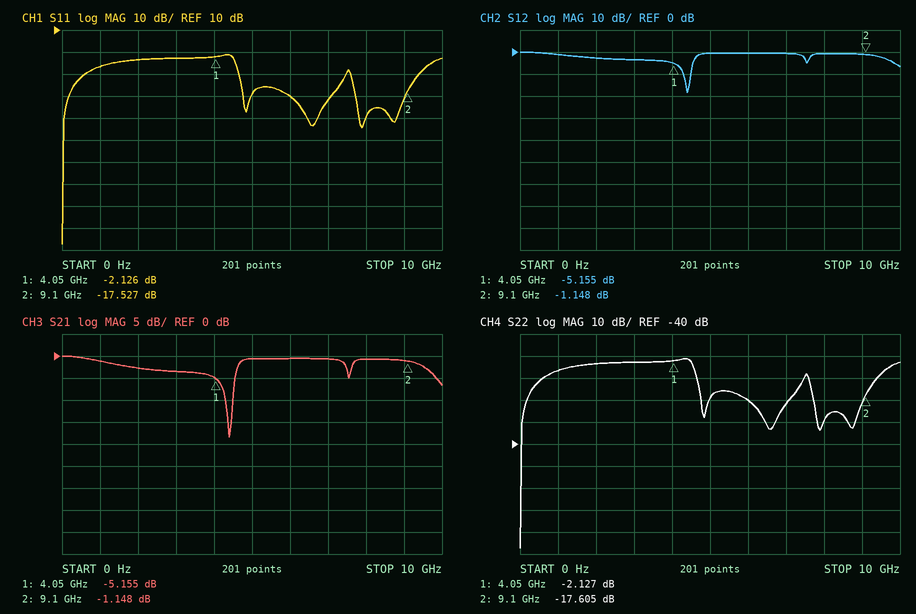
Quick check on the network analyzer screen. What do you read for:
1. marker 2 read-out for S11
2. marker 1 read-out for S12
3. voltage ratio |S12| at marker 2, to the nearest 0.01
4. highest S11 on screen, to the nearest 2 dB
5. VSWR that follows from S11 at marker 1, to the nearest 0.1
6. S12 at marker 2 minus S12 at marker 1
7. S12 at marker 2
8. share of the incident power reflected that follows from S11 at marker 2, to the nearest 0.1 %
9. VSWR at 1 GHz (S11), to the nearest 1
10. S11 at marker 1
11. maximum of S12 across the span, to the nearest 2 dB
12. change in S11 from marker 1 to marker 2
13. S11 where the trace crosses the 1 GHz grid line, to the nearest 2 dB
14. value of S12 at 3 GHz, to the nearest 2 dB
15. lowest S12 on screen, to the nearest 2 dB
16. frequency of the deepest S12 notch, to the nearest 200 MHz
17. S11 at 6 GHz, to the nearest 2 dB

-17.527 dB
-5.155 dB
0.88
-2 dB
8.2
4.007 dB
-1.148 dB
1.8 %
3
-2.126 dB
0 dB
-15.401 dB
-6 dB
-4 dB
-18 dB
4.4 GHz
-20 dB
